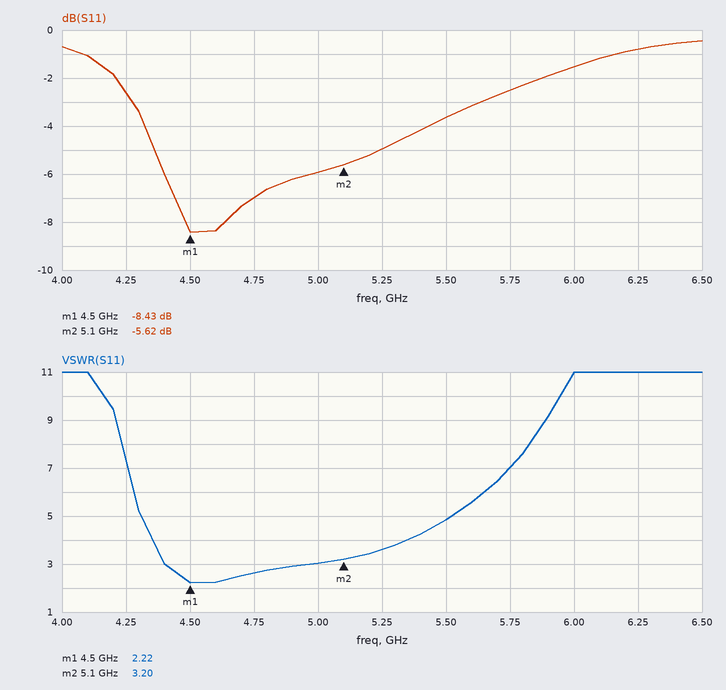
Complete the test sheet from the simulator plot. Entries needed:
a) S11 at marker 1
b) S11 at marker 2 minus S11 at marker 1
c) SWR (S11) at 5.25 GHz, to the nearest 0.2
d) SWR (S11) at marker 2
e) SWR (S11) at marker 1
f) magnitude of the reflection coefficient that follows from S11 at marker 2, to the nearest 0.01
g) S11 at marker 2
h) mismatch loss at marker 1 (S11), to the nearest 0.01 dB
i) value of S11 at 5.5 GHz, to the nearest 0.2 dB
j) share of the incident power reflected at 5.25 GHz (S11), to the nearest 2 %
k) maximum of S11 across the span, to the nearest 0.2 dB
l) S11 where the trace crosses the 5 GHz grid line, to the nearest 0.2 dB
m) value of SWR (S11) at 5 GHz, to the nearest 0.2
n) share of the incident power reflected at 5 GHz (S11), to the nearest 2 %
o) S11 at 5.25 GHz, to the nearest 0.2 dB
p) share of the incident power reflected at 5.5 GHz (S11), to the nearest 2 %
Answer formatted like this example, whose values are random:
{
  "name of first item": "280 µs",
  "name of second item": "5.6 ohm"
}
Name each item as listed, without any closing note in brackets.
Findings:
{
  "S11 at marker 1": "-8.43 dB",
  "S11 at marker 2 minus S11 at marker 1": "2.81 dB",
  "SWR (S11) at 5.25 GHz, to the nearest 0.2": "3.6",
  "SWR (S11) at marker 2": "3.20",
  "SWR (S11) at marker 1": "2.22",
  "magnitude of the reflection coefficient that follows from S11 at marker 2, to the nearest 0.01": "0.52",
  "S11 at marker 2": "-5.62 dB",
  "mismatch loss at marker 1 (S11), to the nearest 0.01 dB": "0.67 dB",
  "value of S11 at 5.5 GHz, to the nearest 0.2 dB": "-3.6 dB",
  "share of the incident power reflected at 5.25 GHz (S11), to the nearest 2 %": "32 %",
  "maximum of S11 across the span, to the nearest 0.2 dB": "-0.4 dB",
  "S11 where the trace crosses the 5 GHz grid line, to the nearest 0.2 dB": "-6.0 dB",
  "value of SWR (S11) at 5 GHz, to the nearest 0.2": "3.0",
  "share of the incident power reflected at 5 GHz (S11), to the nearest 2 %": "26 %",
  "S11 at 5.25 GHz, to the nearest 0.2 dB": "-5.0 dB",
  "share of the incident power reflected at 5.5 GHz (S11), to the nearest 2 %": "44 %"
}
